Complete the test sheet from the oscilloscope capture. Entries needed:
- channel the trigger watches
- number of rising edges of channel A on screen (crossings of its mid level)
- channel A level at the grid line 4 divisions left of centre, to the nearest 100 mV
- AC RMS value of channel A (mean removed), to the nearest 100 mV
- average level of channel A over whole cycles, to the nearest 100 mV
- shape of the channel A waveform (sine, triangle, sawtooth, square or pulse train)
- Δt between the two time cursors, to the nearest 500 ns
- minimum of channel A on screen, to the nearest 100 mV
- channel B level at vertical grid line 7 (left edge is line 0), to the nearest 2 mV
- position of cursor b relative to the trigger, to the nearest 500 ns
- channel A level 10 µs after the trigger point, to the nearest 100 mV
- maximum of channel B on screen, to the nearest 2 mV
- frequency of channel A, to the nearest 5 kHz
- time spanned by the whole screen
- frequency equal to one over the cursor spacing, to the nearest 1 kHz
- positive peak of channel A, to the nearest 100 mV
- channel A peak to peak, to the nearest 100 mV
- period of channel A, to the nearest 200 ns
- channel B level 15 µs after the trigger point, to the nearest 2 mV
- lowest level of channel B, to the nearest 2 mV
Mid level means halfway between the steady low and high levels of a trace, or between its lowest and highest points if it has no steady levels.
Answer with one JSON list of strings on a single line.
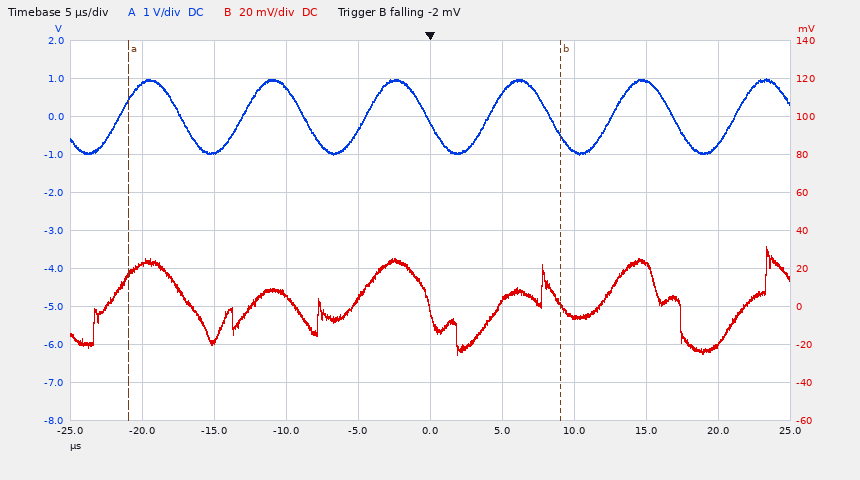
["channel B", "6", "900 mV", "700 mV", "0.0 V", "sine", "30.0 µs", "-1.0 V", "-6 mV", "+9.0 µs", "-900 mV", "32 mV", "115 kHz", "50 µs", "33 kHz", "1.0 V", "2.0 V", "8.6 µs", "22 mV", "-26 mV"]
